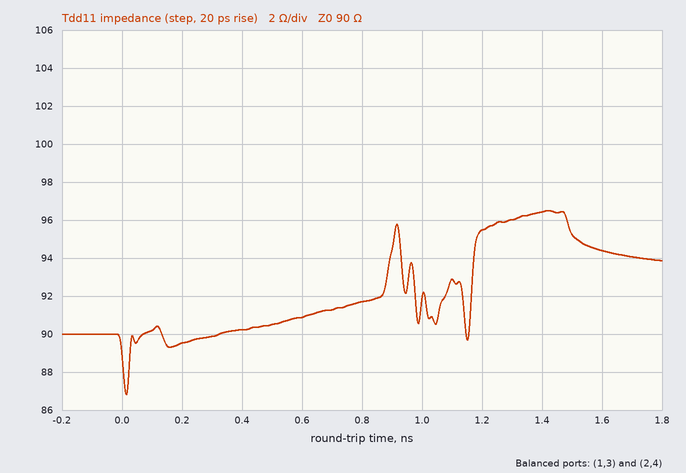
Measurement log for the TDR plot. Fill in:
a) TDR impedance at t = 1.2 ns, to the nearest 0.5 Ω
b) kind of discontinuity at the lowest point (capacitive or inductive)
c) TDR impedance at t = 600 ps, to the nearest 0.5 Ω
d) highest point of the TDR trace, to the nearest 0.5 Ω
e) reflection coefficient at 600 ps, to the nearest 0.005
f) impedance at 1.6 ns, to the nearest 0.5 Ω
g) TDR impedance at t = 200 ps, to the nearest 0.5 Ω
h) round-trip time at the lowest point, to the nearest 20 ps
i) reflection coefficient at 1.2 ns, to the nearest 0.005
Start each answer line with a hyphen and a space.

- 95.5 Ω
- capacitive
- 91.0 Ω
- 96.5 Ω
- +0.005
- 94.5 Ω
- 89.5 Ω
- 20 ps
- +0.030
